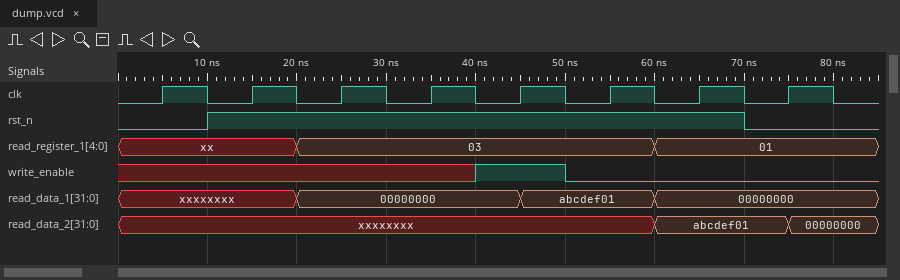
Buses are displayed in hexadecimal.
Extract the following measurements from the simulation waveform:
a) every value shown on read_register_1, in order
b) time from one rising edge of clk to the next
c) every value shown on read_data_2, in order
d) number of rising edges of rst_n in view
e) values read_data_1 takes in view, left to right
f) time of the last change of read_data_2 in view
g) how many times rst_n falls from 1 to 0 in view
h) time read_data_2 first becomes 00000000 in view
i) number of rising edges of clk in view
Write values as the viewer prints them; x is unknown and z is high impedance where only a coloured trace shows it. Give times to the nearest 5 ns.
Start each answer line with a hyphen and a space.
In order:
- xx, 03, 01
- 10 ns
- xxxxxxxx, abcdef01, 00000000
- 1
- xxxxxxxx, 00000000, abcdef01, 00000000
- 75 ns
- 1
- 75 ns
- 8
